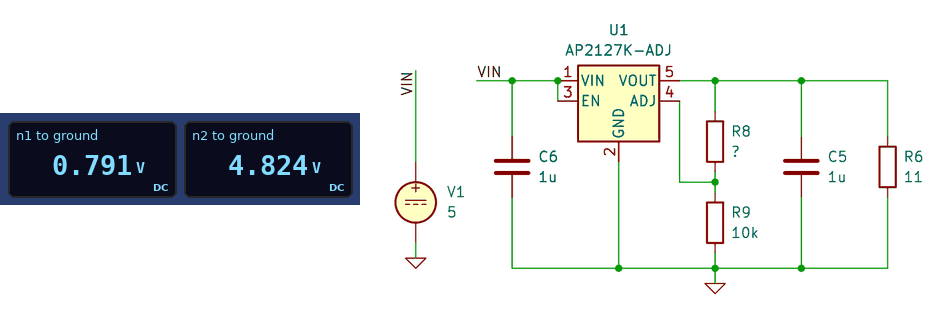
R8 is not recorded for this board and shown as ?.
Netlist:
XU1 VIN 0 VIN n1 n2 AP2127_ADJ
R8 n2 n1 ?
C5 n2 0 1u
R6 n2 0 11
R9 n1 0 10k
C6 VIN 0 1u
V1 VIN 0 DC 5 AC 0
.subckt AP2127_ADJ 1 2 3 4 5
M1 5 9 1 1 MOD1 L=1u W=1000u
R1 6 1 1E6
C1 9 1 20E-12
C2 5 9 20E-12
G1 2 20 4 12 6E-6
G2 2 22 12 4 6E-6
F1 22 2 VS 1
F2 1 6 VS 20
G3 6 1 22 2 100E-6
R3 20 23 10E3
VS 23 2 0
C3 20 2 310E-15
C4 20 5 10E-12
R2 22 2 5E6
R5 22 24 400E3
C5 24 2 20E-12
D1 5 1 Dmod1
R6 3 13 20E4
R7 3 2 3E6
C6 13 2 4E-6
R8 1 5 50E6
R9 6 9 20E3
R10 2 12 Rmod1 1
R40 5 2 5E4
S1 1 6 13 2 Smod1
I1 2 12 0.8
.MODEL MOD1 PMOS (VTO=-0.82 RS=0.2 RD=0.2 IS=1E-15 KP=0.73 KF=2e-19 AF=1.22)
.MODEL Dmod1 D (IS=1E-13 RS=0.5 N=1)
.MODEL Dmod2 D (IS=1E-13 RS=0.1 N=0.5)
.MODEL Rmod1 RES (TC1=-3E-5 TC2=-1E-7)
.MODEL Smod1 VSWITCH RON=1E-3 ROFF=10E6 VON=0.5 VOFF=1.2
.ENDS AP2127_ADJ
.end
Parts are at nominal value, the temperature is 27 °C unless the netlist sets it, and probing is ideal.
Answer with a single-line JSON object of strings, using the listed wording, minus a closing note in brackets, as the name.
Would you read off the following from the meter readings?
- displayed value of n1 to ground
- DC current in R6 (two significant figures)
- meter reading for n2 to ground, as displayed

{"displayed value of n1 to ground": "0.791 V", "DC current in R6": "440 mA", "meter reading for n2 to ground, as displayed": "4.824 V"}
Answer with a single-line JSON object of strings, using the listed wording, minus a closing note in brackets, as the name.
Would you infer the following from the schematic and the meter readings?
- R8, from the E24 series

{"R8, from the E24 series": "51 kΩ"}
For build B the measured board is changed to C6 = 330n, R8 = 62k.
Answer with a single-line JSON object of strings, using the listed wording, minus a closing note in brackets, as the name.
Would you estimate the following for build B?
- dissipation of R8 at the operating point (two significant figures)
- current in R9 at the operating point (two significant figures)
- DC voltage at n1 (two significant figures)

{"dissipation of R8 at the operating point": "280 µW", "current in R9 at the operating point": "67 µA", "DC voltage at n1": "670 mV"}
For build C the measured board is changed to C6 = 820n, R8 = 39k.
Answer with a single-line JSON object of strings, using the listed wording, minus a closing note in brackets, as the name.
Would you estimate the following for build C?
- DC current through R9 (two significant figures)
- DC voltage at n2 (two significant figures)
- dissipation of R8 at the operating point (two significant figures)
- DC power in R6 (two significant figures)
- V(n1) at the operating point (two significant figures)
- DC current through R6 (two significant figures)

{"DC current through R9": "80 µA", "DC voltage at n2": "3.9 V", "dissipation of R8 at the operating point": "250 µW", "DC power in R6": "1.4 W", "V(n1) at the operating point": "800 mV", "DC current through R6": "360 mA"}
